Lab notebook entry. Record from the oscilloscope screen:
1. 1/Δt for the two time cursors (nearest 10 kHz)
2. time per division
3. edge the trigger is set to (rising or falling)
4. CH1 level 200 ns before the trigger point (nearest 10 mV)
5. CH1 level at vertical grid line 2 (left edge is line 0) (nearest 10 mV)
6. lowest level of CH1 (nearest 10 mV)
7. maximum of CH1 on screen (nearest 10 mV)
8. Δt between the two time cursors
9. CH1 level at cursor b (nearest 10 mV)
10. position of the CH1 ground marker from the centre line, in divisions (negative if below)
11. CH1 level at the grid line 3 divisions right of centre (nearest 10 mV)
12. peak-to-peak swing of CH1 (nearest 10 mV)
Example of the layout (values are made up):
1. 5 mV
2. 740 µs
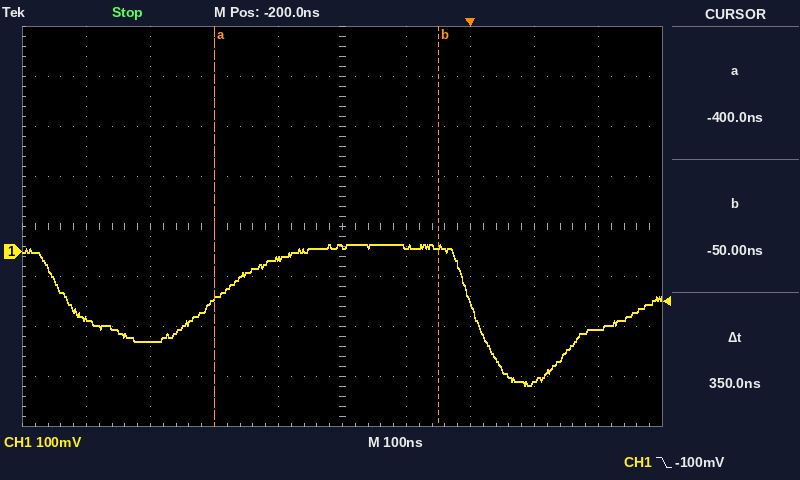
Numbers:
1. 2.86 MHz
2. 100 ns
3. falling
4. 10 mV
5. -180 mV
6. -270 mV
7. 10 mV
8. 350 ns
9. 10 mV
10. -0.5 div
11. -260 mV
12. 280 mV
